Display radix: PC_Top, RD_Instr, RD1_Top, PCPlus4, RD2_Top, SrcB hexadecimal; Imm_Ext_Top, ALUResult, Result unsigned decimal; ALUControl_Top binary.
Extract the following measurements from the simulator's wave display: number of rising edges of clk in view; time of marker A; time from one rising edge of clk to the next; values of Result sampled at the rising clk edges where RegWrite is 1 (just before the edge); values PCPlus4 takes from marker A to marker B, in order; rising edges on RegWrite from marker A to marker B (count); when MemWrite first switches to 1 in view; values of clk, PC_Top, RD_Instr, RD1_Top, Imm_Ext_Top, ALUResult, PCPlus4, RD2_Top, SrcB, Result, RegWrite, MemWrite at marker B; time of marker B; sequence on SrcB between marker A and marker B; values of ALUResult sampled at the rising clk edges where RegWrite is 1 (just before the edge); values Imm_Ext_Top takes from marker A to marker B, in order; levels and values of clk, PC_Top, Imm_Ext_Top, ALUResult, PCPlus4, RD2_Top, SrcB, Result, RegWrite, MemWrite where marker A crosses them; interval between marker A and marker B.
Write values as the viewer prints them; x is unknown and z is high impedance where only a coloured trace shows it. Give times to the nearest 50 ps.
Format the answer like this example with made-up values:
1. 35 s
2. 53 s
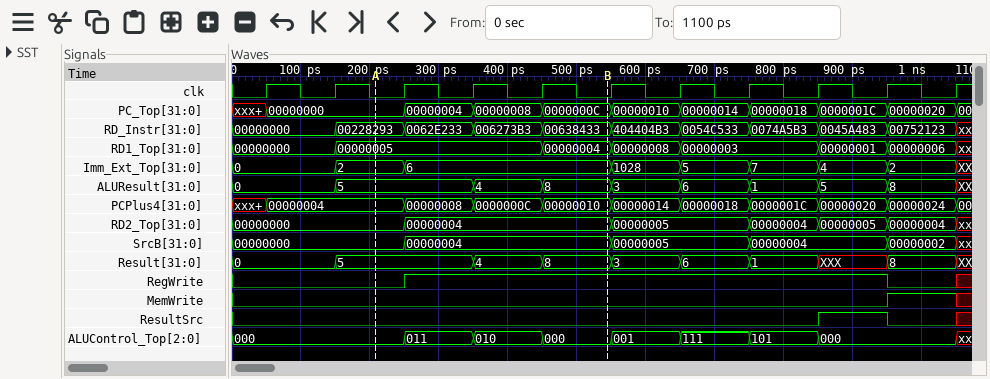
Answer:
1. 11
2. 200 ps
3. 100 ps
4. 5, 4, 8, 3, 6, 1, XXX
5. 00000004, 00000008, 0000000C, 00000010
6. 1
7. 950 ps
8. clk=0, PC_Top=0000000C, RD_Instr=00638433, RD1_Top=00000004, Imm_Ext_Top=6, ALUResult=8, PCPlus4=00000010, RD2_Top=00000004, SrcB=00000004, Result=8, RegWrite=1, MemWrite=0
9. 550 ps
10. 00000000, 00000004
11. 5, 4, 8, 3, 6, 1, 5
12. 2, 6
13. clk=0, PC_Top=00000000, Imm_Ext_Top=2, ALUResult=5, PCPlus4=00000004, RD2_Top=00000000, SrcB=00000000, Result=5, RegWrite=0, MemWrite=0
14. 350 ps
